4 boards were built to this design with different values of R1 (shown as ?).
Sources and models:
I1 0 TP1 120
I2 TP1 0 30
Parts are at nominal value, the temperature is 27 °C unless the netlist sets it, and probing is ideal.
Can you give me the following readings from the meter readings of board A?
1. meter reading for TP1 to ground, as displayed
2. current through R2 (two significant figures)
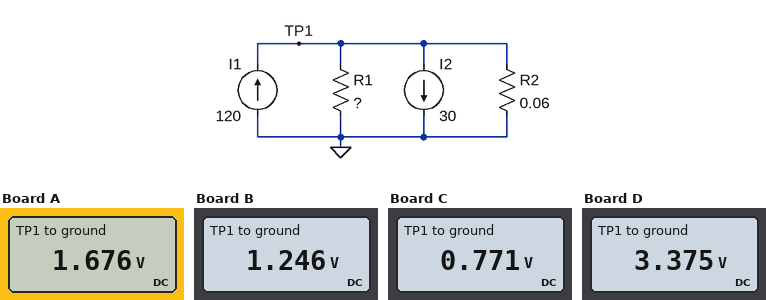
1.676 V
28 A
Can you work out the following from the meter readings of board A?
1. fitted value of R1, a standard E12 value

0.027 Ω
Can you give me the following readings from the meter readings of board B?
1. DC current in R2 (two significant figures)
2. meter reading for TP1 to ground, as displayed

21 A
1.246 V
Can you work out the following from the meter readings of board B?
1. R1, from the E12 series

0.018 Ω
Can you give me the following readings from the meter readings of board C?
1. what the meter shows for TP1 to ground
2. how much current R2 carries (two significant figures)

0.771 V
13 A
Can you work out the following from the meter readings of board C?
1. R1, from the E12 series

0.01 Ω
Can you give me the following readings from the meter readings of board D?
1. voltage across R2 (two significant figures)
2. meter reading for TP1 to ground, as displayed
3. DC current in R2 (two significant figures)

3.4 V
3.375 V
56 A
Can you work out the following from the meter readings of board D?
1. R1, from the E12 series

0.1 Ω
